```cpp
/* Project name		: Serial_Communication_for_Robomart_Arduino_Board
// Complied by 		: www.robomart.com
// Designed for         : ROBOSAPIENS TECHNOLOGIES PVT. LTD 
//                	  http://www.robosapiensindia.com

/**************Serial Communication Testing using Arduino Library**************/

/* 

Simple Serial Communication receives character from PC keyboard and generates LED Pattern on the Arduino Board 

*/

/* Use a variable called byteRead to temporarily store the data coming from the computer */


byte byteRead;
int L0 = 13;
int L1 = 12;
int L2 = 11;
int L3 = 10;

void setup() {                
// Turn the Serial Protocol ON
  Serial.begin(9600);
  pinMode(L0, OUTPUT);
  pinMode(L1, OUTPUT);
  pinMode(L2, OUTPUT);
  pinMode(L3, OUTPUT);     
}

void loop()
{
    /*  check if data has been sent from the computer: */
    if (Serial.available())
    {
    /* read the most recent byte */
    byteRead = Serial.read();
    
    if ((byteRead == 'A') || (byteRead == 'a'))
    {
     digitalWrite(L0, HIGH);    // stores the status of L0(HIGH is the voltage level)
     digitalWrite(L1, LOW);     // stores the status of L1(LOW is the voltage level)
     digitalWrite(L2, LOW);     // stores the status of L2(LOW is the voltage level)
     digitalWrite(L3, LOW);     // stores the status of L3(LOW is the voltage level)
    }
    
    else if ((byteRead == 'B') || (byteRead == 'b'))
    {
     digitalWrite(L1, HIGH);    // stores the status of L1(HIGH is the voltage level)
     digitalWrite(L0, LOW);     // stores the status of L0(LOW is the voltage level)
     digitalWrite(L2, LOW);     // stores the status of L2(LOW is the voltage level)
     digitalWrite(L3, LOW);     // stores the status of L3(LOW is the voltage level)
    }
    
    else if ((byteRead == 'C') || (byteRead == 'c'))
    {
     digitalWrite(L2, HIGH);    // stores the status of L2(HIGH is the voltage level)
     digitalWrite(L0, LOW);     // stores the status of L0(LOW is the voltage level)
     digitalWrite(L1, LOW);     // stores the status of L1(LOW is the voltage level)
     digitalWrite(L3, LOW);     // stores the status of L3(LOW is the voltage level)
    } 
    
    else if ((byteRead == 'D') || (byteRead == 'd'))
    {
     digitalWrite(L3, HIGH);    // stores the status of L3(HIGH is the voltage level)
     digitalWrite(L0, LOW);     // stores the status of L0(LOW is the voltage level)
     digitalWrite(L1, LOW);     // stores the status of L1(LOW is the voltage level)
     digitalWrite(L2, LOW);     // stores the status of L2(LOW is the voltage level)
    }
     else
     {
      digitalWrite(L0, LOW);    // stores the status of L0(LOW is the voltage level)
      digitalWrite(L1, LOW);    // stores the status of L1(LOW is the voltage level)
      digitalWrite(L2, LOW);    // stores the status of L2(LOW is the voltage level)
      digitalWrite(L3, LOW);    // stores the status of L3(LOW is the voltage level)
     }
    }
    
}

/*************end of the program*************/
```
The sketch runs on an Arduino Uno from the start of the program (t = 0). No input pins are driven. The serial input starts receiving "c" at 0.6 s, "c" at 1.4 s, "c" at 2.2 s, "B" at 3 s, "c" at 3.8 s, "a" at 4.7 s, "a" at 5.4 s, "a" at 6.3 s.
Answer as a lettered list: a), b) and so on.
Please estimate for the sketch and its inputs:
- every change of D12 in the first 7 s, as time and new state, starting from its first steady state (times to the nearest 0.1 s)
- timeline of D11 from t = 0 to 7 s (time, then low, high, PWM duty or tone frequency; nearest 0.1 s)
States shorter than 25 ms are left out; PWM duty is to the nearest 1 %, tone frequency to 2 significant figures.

a) 0 s low; 3 s high; 3.8 s low
b) 0 s low; 0.6 s high; 3 s low; 3.8 s high; 4.7 s low
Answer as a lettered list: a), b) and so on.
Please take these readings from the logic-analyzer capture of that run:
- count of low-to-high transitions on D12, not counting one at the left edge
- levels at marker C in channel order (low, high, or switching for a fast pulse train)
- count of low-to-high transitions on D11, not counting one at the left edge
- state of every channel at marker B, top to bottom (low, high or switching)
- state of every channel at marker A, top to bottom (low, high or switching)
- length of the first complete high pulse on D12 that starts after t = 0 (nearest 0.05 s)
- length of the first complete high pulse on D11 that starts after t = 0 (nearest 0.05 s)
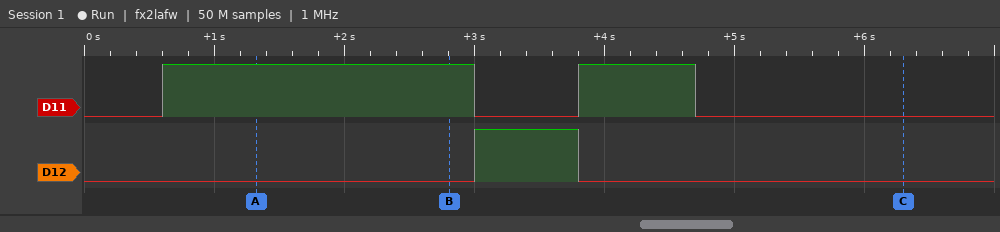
a) 1
b) D11 low, D12 low
c) 2
d) D11 high, D12 low
e) D11 high, D12 low
f) 0.80 s
g) 2.40 s
